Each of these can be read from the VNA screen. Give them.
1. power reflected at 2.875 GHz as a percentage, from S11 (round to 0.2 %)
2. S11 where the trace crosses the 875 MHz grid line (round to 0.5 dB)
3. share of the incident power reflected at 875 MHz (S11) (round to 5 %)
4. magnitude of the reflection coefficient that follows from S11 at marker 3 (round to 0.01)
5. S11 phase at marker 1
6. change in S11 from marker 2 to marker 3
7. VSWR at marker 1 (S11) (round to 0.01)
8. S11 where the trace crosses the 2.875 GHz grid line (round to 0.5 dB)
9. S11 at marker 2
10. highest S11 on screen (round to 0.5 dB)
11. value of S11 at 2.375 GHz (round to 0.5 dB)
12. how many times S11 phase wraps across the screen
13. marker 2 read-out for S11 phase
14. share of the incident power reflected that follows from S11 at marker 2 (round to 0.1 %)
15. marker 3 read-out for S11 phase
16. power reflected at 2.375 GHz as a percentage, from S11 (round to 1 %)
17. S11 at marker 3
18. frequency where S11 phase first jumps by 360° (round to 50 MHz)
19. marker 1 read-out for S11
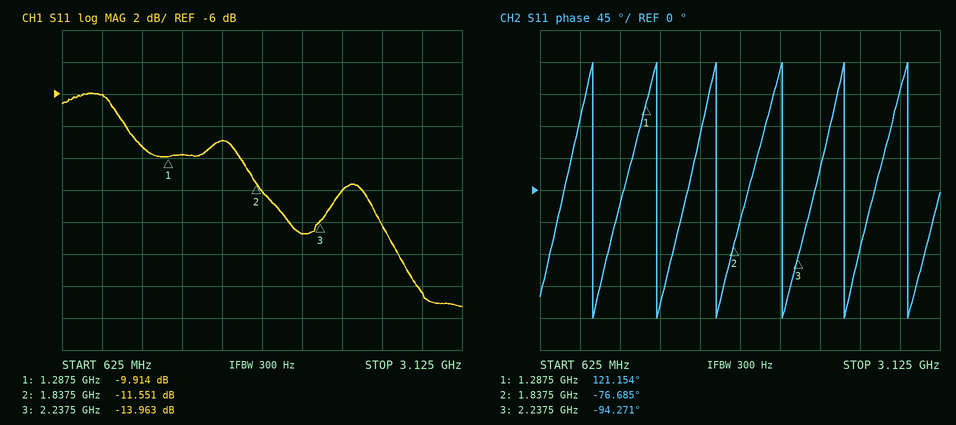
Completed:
1.4 %
-6.0 dB
25 %
0.20
121.154°
-2.412 dB
1.94
-18.5 dB
-11.551 dB
-6.0 dB
-12.0 dB
6
-76.685°
7.0 %
-94.271°
6 %
-13.963 dB
950 MHz
-9.914 dB
